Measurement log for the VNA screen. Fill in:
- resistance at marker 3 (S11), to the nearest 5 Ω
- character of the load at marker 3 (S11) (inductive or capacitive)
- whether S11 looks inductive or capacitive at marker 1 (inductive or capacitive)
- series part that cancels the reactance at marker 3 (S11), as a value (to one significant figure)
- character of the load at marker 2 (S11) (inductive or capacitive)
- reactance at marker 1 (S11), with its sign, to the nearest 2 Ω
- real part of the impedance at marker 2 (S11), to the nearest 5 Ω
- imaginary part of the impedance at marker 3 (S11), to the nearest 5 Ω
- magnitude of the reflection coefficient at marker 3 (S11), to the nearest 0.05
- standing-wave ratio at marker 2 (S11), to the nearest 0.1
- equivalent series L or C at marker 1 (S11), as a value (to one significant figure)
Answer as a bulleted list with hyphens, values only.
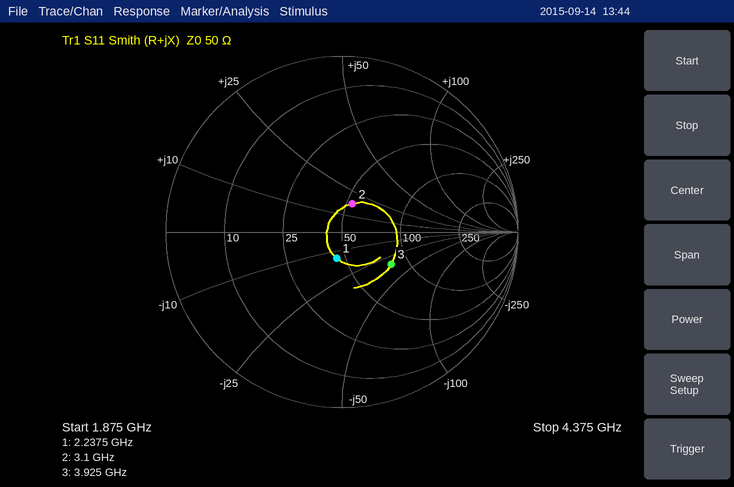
- 80 Ω
- capacitive
- capacitive
- 1 nH
- inductive
- -14 Ω
- 55 Ω
- -35 Ω
- 0.35
- 1.4
- 5 pF
